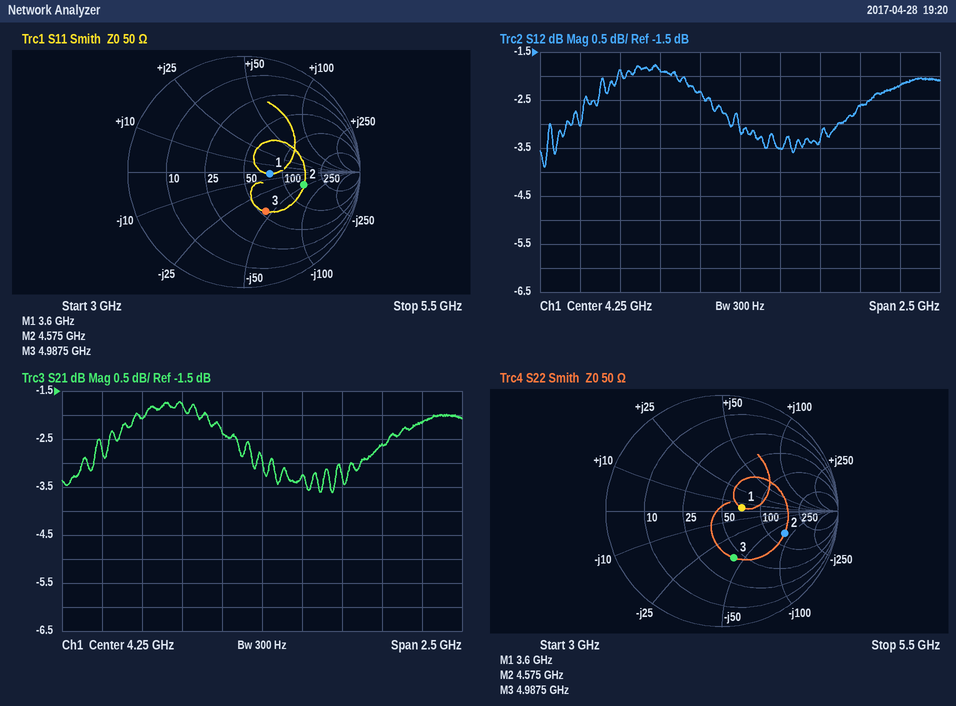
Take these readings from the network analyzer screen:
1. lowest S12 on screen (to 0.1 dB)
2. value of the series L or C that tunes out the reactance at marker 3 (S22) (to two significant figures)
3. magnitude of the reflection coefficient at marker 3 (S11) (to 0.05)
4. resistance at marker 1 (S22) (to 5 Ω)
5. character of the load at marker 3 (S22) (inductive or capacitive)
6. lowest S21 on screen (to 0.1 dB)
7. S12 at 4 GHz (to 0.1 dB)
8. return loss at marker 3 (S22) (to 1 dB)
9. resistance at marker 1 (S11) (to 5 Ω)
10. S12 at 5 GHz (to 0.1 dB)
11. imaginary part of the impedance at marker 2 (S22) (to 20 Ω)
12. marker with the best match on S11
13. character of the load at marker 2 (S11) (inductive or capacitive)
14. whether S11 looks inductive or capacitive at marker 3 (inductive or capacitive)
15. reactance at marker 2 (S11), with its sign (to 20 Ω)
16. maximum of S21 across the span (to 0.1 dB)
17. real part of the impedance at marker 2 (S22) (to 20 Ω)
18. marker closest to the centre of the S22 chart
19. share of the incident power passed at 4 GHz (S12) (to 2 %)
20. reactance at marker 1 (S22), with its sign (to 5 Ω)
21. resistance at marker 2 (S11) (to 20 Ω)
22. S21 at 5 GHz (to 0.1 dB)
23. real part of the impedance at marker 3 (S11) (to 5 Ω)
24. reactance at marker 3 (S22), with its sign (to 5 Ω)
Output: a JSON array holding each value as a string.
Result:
["-3.9 dB", "1.3 nH", "0.40", "70 Ω", "capacitive", "-3.6 dB", "-2.3 dB", "8 dB", "80 Ω", "-2.6 dB", "-80 Ω", "marker 1", "capacitive", "capacitive", "-40 Ω", "-1.7 dB", "140 Ω", "marker 1", "58 %", "+5 Ω", "140 Ω", "-2.6 dB", "55 Ω", "-40 Ω"]
